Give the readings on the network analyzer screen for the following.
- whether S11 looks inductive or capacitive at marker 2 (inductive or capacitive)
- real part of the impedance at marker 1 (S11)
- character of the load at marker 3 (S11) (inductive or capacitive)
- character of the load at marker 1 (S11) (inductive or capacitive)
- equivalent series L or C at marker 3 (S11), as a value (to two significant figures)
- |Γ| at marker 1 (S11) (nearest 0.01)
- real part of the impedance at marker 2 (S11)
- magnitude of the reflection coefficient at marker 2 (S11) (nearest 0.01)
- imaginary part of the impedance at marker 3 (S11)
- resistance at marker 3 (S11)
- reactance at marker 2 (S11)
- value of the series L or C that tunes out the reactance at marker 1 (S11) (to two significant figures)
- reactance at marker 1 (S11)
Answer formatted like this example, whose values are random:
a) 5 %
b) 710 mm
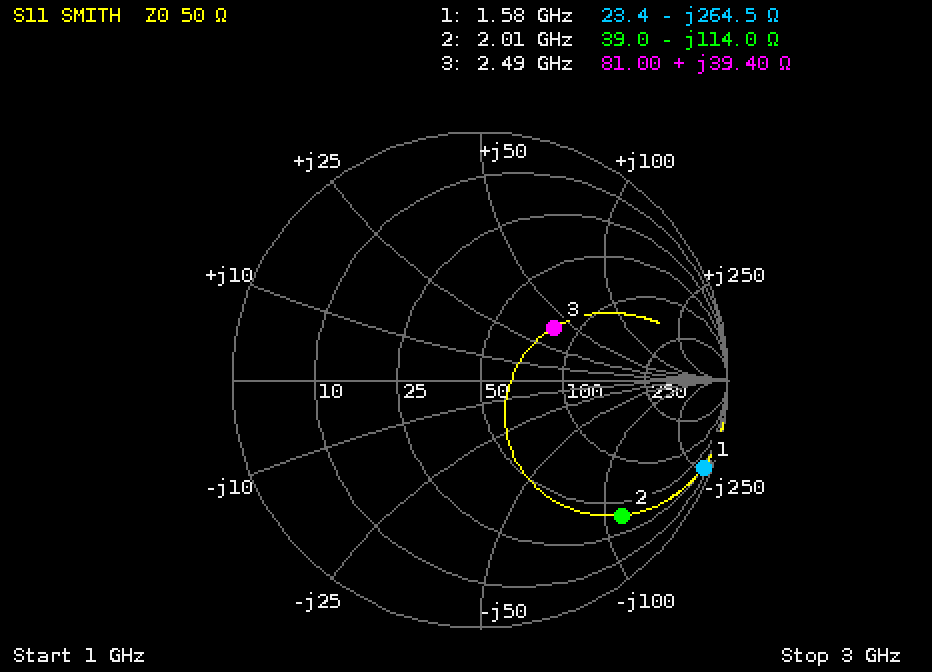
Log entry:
a) capacitive
b) 23.4 Ω
c) inductive
d) capacitive
e) 2.5 nH
f) 0.97
g) 39.0 Ω
h) 0.79
i) +39.40 Ω
j) 81.00 Ω
k) -114.0 Ω
l) 27 nH
m) -264.5 Ω
